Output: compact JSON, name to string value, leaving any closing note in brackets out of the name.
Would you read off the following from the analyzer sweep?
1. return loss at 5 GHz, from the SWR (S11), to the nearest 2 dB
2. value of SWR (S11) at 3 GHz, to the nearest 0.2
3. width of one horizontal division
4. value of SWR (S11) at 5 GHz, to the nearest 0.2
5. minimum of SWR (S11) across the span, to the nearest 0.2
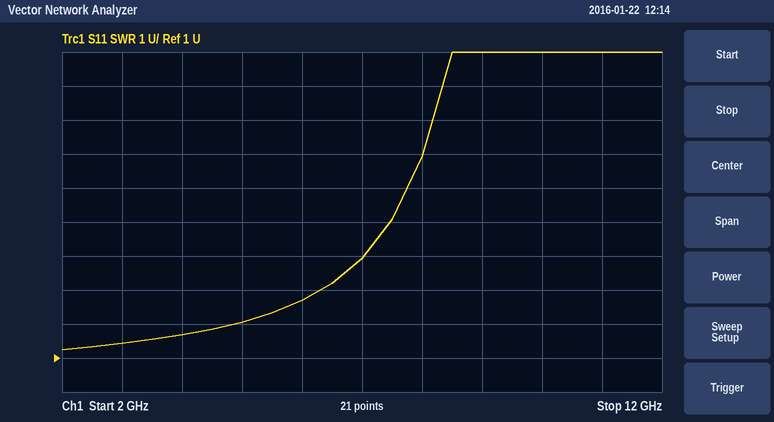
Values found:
{"return loss at 5 GHz, from the SWR (S11), to the nearest 2 dB": "10 dB", "value of SWR (S11) at 3 GHz, to the nearest 0.2": "1.4", "width of one horizontal division": "1 GHz", "value of SWR (S11) at 5 GHz, to the nearest 0.2": "2.0", "minimum of SWR (S11) across the span, to the nearest 0.2": "1.2"}
